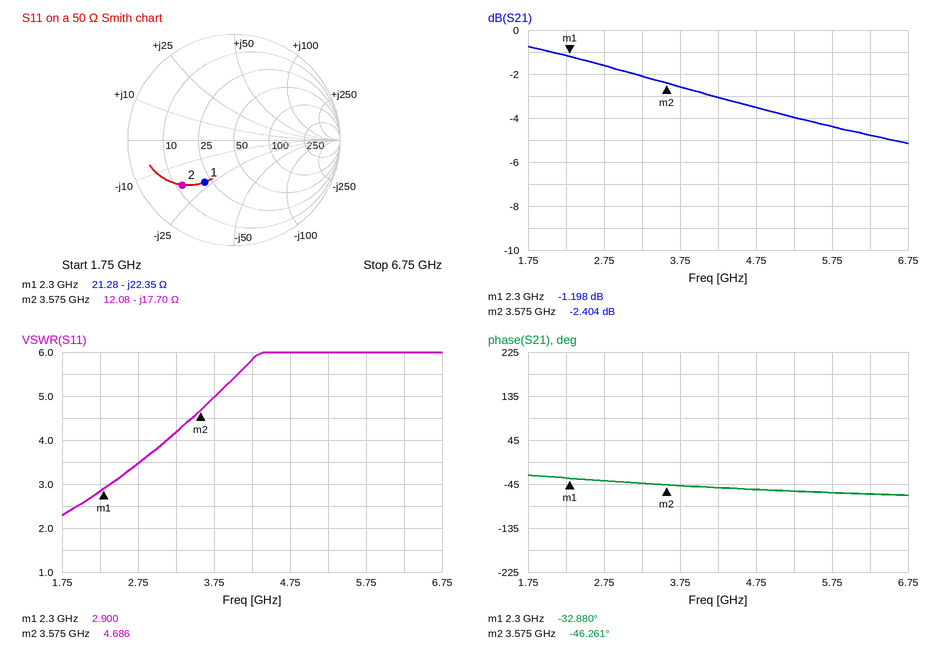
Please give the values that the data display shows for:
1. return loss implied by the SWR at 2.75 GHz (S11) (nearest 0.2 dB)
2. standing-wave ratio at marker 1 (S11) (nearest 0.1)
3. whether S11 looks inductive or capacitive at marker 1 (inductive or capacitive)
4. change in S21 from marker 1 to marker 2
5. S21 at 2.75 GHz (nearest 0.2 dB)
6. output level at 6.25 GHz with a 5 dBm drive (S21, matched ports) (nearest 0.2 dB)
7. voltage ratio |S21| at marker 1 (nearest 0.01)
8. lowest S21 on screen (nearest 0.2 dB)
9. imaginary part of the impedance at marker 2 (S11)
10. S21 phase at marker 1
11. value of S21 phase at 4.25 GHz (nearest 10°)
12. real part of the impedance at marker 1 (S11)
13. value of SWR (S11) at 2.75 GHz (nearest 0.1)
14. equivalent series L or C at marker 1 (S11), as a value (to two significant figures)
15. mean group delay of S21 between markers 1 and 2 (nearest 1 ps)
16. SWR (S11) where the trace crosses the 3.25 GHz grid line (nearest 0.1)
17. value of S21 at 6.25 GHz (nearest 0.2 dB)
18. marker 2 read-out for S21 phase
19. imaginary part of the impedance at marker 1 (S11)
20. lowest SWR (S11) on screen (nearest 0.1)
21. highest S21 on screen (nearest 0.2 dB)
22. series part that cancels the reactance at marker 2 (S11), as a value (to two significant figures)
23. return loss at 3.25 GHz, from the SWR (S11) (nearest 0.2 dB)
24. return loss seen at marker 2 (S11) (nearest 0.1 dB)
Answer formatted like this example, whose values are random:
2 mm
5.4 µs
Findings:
5.2 dB
2.9
capacitive
-1.206 dB
-1.6 dB
0.2 dBm
0.87
-5.2 dB
-17.70 Ω
-32.880°
-50°
21.28 Ω
3.5
3.1 pF
29 ps
4.2
-4.8 dB
-46.261°
-22.35 Ω
2.3
-0.8 dB
790 pH
4.2 dB
3.8 dB
